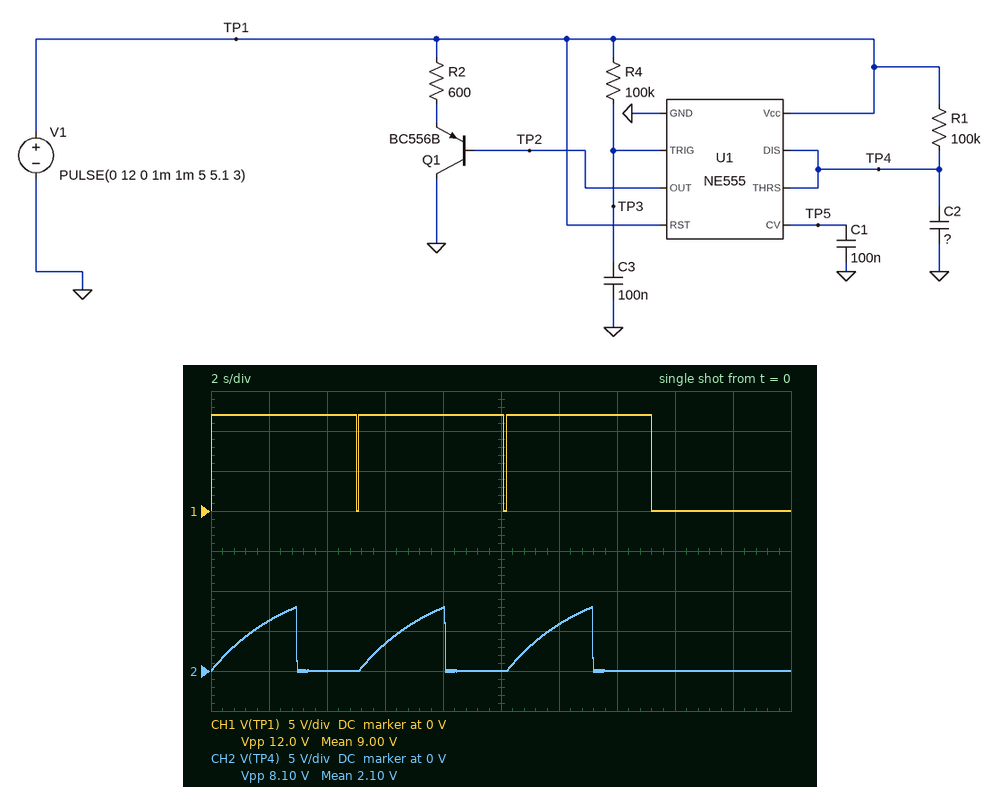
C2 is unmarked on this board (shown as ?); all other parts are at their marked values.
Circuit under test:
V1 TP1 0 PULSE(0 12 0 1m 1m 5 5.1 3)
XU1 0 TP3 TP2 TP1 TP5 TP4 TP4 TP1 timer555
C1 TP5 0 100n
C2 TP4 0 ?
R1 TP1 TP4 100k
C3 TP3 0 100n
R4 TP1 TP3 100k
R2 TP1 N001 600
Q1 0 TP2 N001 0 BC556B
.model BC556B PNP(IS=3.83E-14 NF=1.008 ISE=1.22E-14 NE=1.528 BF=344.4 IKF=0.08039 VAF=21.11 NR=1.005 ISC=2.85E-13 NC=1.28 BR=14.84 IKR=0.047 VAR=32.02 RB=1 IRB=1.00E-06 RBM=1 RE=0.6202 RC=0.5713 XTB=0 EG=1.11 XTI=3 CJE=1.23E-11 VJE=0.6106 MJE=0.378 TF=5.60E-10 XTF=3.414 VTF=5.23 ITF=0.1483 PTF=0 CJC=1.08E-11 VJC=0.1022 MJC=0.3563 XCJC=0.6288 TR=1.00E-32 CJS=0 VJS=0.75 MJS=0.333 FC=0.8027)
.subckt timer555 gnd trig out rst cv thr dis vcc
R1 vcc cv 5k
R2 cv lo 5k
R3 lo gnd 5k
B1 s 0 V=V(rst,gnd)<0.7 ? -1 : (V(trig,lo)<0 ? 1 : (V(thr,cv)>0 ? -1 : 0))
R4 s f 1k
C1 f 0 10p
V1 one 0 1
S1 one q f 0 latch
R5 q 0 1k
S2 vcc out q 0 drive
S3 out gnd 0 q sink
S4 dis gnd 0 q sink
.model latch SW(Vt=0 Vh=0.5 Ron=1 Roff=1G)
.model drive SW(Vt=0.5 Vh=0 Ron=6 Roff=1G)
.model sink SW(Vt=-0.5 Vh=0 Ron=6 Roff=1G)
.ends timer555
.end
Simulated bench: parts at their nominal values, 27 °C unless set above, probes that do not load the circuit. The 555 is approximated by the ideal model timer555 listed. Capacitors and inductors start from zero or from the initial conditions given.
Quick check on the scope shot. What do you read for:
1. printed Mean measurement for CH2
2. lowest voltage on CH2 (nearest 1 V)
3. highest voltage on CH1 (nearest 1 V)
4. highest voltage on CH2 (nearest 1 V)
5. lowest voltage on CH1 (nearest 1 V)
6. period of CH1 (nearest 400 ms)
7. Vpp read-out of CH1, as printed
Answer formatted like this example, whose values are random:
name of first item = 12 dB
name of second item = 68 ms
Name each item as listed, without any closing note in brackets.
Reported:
printed Mean measurement for CH2 = 2.10 V
lowest voltage on CH2 = 0 V
highest voltage on CH1 = 12 V
highest voltage on CH2 = 8 V
lowest voltage on CH1 = 0 V
period of CH1 = 5.2 s
Vpp read-out of CH1, as printed = 12.0 V
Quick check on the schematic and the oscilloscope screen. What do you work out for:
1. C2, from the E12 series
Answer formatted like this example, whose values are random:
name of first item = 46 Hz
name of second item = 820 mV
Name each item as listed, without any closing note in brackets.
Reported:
C2, from the E12 series = 27 µF
